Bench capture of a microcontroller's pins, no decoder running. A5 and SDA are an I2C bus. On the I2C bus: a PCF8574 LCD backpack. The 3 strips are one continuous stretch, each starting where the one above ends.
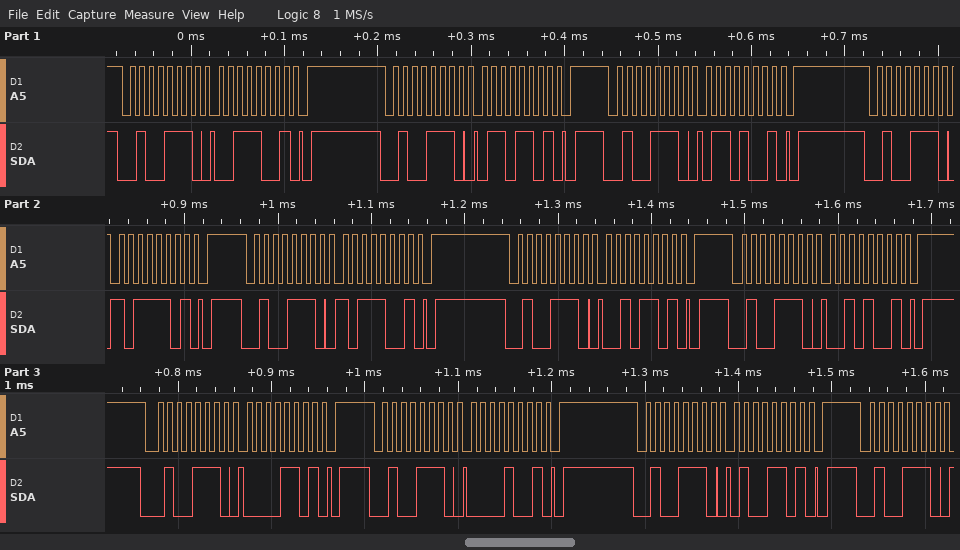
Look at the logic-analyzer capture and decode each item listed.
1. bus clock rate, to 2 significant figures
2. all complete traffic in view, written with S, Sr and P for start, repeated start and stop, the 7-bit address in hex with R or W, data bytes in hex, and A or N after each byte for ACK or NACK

100 kHz
S 27W A 39 A P S 27W A 6D A P S 27W A 69 A P S 27W A BD A P S 27W A B9 A P S 27W A 2D A P S 27W A 29 A P S 27W A 0D A P S 27W A 09 A P S 27W A 4D A P S 27W A
